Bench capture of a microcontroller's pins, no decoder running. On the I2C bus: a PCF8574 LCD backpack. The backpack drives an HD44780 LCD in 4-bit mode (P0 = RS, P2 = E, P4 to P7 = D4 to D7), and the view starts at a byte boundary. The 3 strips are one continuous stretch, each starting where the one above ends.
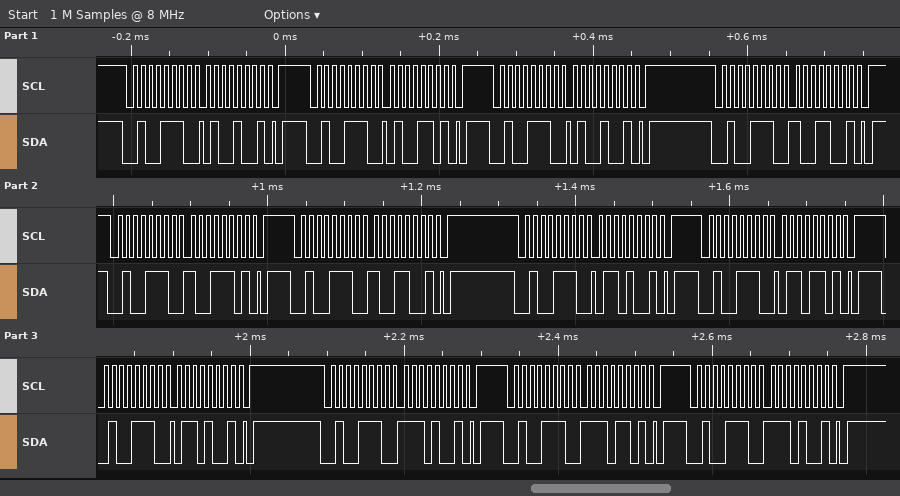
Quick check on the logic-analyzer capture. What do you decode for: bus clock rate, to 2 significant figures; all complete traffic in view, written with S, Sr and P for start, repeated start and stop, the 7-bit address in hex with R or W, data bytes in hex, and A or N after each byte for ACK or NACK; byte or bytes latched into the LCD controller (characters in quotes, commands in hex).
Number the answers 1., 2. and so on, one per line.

1. 100 kHz
2. S 27W A 49 A P S 27W A 4D A P S 27W A 49 A P S 27W A 99 A P S 27W A 9D A P S 27W A 99 A P S 27W A 69 A P S 27W A 6D A P S 27W A 69 A P S 27W A E9 A P S 27W A ED A P S 27W A E9 A P
3. 'I' 'n'
